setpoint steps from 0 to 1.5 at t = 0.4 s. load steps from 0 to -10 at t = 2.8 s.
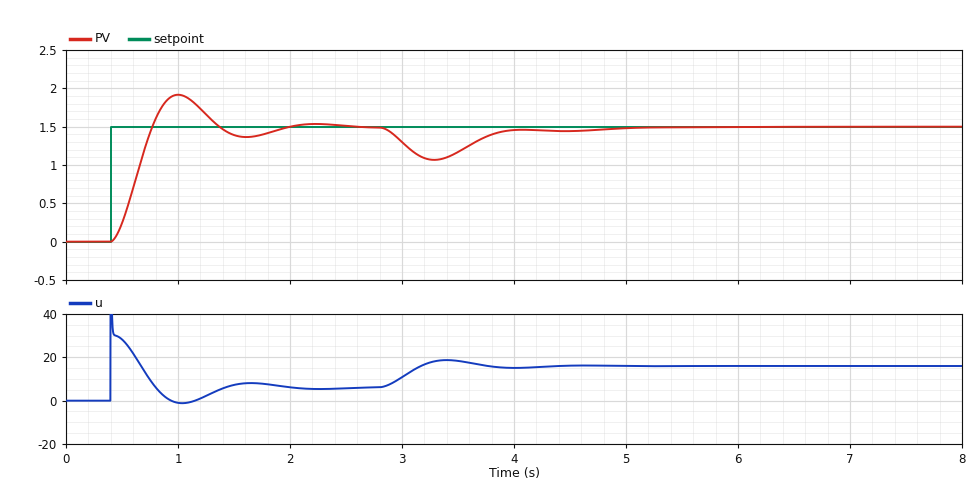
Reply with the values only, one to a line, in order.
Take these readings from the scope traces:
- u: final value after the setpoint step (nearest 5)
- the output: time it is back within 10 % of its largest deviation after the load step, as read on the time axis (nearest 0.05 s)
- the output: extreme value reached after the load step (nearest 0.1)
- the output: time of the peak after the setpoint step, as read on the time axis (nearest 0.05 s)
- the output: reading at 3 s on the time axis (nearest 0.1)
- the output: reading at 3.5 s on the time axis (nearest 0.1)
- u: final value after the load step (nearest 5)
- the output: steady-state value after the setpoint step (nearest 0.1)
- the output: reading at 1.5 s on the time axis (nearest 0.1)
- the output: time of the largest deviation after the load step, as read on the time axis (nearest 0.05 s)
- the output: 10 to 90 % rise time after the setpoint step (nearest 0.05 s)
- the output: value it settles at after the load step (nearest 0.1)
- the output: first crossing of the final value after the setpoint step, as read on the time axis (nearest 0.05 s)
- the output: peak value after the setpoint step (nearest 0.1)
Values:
5
4.75 s
1.1
1.00 s
1.3
1.2
15
1.5
1.4
3.30 s
0.25 s
1.5
0.75 s
1.9
